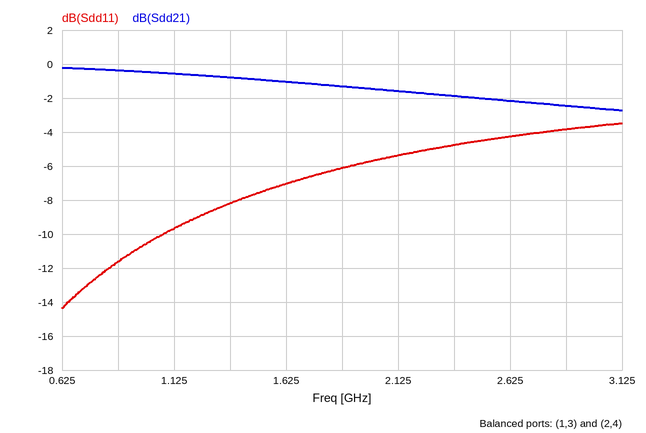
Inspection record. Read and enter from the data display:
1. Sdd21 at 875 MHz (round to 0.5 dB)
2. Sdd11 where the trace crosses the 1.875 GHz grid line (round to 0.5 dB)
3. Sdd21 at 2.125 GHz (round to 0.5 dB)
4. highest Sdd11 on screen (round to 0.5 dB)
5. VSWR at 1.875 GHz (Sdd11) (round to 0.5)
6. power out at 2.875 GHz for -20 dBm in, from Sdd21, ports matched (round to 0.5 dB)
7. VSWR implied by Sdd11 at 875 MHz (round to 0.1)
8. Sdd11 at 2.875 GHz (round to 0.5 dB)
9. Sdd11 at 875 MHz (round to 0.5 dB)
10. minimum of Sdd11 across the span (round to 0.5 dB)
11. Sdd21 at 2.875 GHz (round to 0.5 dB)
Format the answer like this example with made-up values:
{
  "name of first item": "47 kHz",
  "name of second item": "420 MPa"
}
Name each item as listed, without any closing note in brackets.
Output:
{
  "Sdd21 at 875 MHz": "-0.5 dB",
  "Sdd11 where the trace crosses the 1.875 GHz grid line": "-6.0 dB",
  "Sdd21 at 2.125 GHz": "-1.5 dB",
  "highest Sdd11 on screen": "-3.5 dB",
  "VSWR at 1.875 GHz (Sdd11)": "3.0",
  "power out at 2.875 GHz for -20 dBm in, from Sdd21, ports matched": "-22.5 dBm",
  "VSWR implied by Sdd11 at 875 MHz": "1.7",
  "Sdd11 at 2.875 GHz": "-4.0 dB",
  "Sdd11 at 875 MHz": "-11.5 dB",
  "minimum of Sdd11 across the span": "-14.5 dB",
  "Sdd21 at 2.875 GHz": "-2.5 dB"
}
